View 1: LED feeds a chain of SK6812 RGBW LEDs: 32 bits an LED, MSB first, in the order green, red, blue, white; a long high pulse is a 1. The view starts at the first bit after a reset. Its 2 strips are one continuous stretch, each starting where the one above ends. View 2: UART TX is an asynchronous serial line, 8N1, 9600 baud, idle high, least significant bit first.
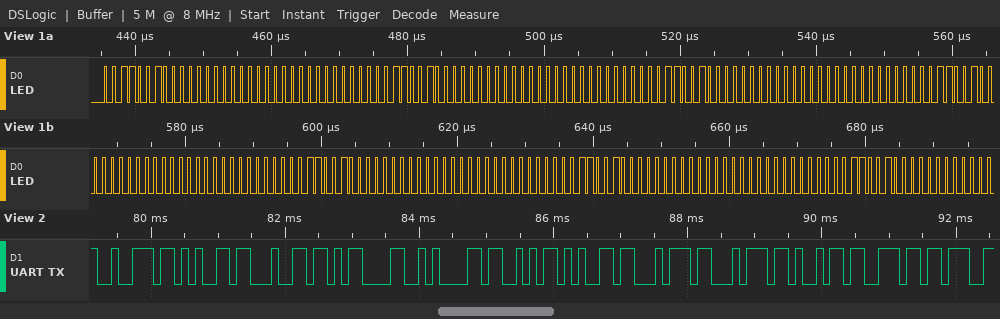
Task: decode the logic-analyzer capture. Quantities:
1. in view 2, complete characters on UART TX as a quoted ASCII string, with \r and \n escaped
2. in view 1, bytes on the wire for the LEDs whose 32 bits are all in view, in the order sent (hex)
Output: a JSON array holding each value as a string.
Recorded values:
["\"red\\r\\nSettin\"", "32 00 00 00 32 00 00 00 32 00 00 00 32 00 00 00 32 00 00 00 32 00 00 00"]
